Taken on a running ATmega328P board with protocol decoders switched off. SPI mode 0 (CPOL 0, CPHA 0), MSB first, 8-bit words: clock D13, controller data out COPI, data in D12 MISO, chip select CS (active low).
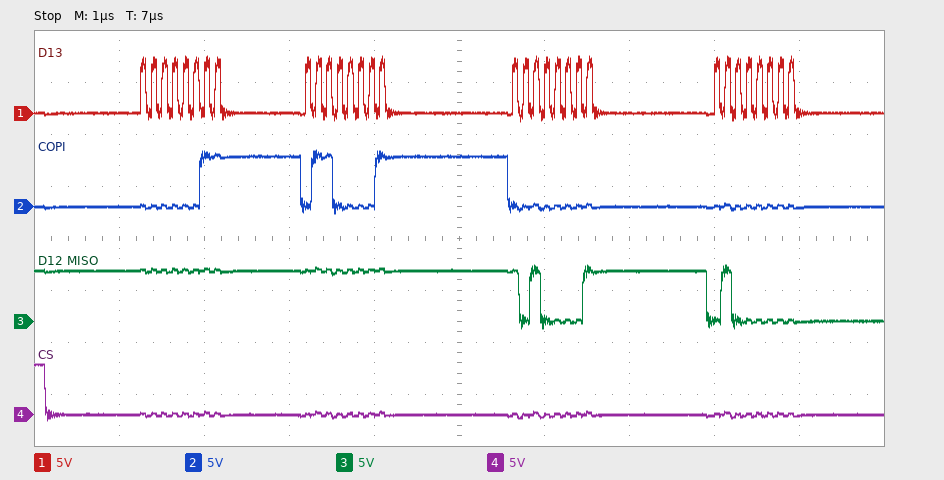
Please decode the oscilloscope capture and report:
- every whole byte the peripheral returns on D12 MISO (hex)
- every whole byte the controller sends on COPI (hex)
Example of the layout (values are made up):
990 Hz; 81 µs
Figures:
FF FF A1 40; 03 61 00 00
